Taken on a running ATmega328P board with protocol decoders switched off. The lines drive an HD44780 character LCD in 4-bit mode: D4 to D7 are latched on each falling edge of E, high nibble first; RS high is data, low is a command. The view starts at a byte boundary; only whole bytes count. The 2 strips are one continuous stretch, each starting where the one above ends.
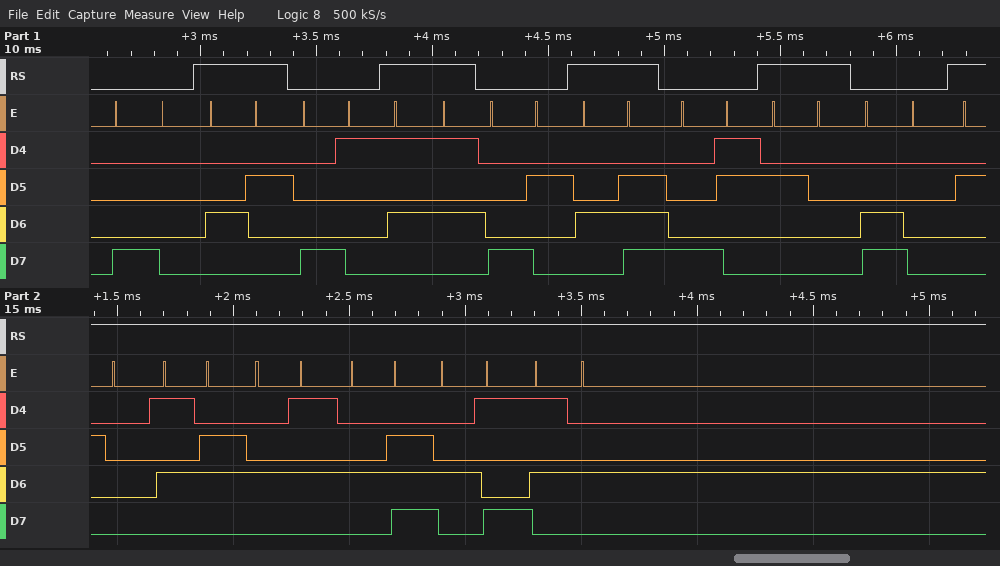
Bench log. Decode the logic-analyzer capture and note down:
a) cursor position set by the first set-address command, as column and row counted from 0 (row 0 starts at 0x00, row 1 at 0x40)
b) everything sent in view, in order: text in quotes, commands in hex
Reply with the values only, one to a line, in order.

column 0, row 0
0x80 "B" 0x81 "U" 0x82 "N" 0x83 " " 0xC0 " VENIT"
